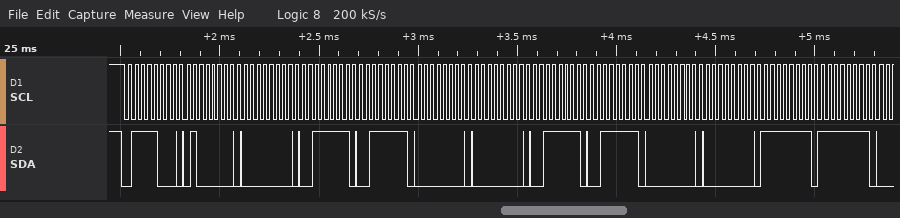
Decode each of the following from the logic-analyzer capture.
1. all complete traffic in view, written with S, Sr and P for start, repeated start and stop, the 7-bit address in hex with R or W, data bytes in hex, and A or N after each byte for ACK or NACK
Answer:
S 3CW A 40 A 00 A 3F A 3F A 00 A 00 A 3F A 3F A 00 A 00 A FF A FF A
